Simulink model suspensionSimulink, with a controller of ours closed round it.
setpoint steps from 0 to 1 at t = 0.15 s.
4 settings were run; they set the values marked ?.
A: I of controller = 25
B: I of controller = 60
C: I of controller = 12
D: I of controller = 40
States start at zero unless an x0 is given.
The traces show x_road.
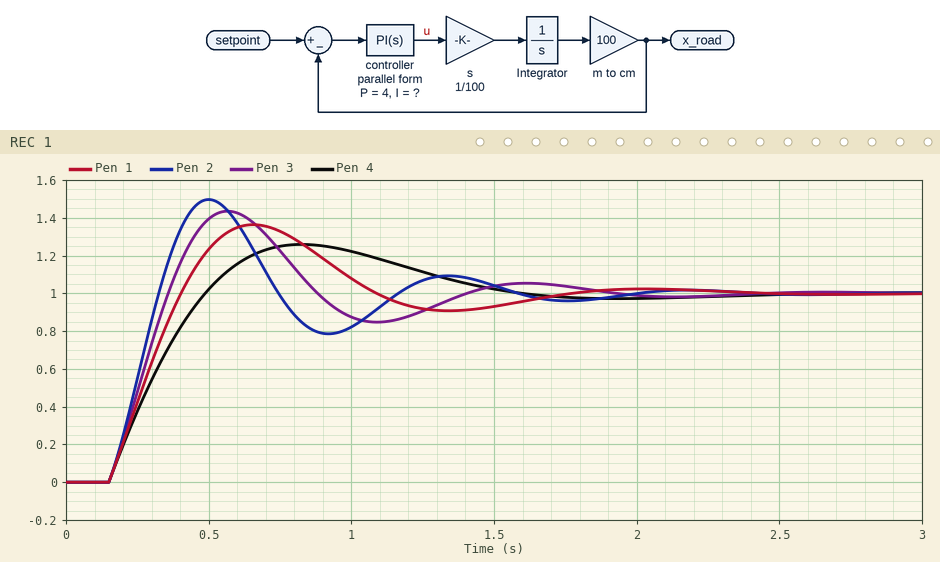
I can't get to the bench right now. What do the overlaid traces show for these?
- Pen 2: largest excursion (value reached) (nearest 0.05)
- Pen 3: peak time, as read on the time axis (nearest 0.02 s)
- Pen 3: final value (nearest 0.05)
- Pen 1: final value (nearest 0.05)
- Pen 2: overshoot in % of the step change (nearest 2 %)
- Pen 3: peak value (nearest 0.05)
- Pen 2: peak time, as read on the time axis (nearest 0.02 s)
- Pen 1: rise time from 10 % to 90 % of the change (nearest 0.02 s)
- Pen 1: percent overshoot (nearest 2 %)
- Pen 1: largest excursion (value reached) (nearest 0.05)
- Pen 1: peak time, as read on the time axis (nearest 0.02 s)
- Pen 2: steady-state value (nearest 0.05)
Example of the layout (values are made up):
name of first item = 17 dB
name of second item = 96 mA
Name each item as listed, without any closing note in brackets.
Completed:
Pen 2: largest excursion (value reached) = 1.50
Pen 3: peak time, as read on the time axis = 0.56 s
Pen 3: final value = 1.00
Pen 1: final value = 1.00
Pen 2: overshoot in % of the step change = 50 %
Pen 3: peak value = 1.45
Pen 2: peak time, as read on the time axis = 0.50 s
Pen 1: rise time from 10 % to 90 % of the change = 0.20 s
Pen 1: percent overshoot = 36 %
Pen 1: largest excursion (value reached) = 1.35
Pen 1: peak time, as read on the time axis = 0.66 s
Pen 2: steady-state value = 1.00
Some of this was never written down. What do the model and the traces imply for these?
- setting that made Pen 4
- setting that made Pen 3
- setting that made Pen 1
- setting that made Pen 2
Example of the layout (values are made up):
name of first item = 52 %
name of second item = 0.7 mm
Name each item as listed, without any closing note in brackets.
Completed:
setting that made Pen 4 = C
setting that made Pen 3 = D
setting that made Pen 1 = A
setting that made Pen 2 = B
